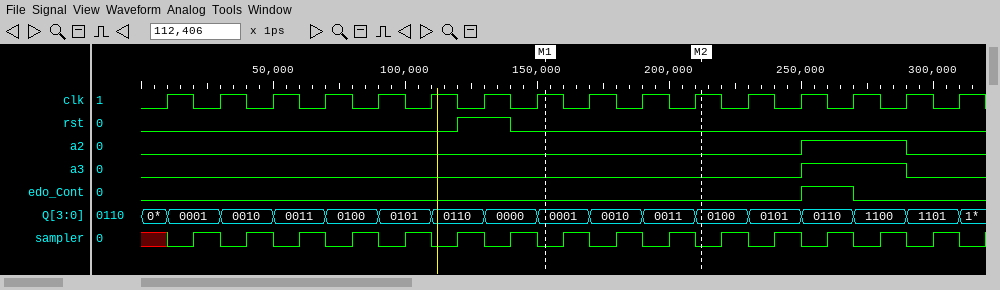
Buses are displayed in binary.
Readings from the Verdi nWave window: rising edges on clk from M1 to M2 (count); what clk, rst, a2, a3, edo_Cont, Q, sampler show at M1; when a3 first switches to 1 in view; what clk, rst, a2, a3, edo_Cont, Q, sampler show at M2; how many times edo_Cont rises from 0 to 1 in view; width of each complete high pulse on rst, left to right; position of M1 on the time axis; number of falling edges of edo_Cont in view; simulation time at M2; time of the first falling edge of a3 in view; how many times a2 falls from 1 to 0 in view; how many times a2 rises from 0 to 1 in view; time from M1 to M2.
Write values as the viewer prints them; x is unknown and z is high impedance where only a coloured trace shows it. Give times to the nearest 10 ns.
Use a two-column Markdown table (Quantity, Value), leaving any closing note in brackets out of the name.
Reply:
| Quantity | Value |
|---|---|
| rising edges on clk from M1 to M2 | 3 |
| what clk, rst, a2, a3, edo_Cont, Q, sampler show at M1 | clk=1, rst=0, a2=0, a3=0, edo_Cont=0, Q=0001, sampler=0 |
| when a3 first switches to 1 in view | 250 ns |
| what clk, rst, a2, a3, edo_Cont, Q, sampler show at M2 | clk=1, rst=0, a2=0, a3=0, edo_Cont=0, Q=0100, sampler=0 |
| how many times edo_Cont rises from 0 to 1 in view | 1 |
| width of each complete high pulse on rst, left to right | 20 ns |
| position of M1 on the time axis | 150 ns |
| number of falling edges of edo_Cont in view | 1 |
| simulation time at M2 | 210 ns |
| time of the first falling edge of a3 in view | 290 ns |
| how many times a2 falls from 1 to 0 in view | 1 |
| how many times a2 rises from 0 to 1 in view | 1 |
| time from M1 to M2 | 60 ns |
